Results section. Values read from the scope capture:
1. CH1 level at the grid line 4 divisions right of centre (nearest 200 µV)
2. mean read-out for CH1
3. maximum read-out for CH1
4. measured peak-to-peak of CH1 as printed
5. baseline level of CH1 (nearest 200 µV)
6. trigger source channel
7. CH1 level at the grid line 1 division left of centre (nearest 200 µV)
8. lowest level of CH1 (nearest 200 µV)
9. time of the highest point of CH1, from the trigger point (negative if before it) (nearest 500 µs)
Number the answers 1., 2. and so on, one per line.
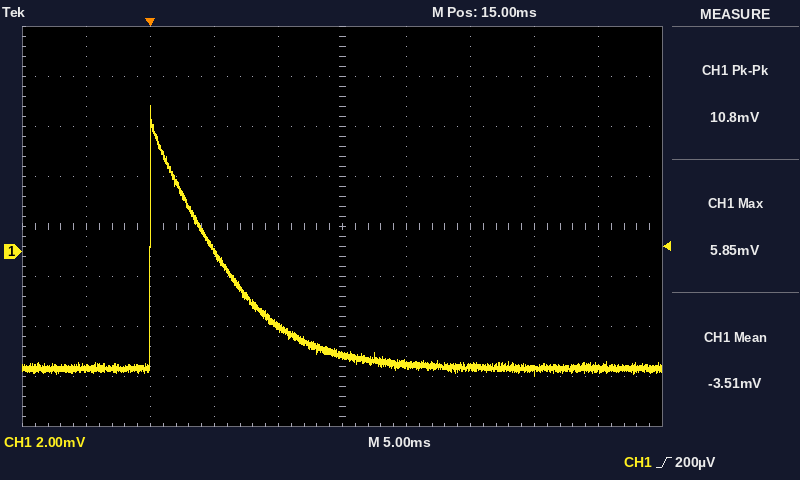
1. -4.6 mV
2. -3.51 mV
3. 5.85 mV
4. 10.8 mV
5. -4.6 mV
6. CH1
7. -3.0 mV
8. -5.0 mV
9. 0.0 ms
